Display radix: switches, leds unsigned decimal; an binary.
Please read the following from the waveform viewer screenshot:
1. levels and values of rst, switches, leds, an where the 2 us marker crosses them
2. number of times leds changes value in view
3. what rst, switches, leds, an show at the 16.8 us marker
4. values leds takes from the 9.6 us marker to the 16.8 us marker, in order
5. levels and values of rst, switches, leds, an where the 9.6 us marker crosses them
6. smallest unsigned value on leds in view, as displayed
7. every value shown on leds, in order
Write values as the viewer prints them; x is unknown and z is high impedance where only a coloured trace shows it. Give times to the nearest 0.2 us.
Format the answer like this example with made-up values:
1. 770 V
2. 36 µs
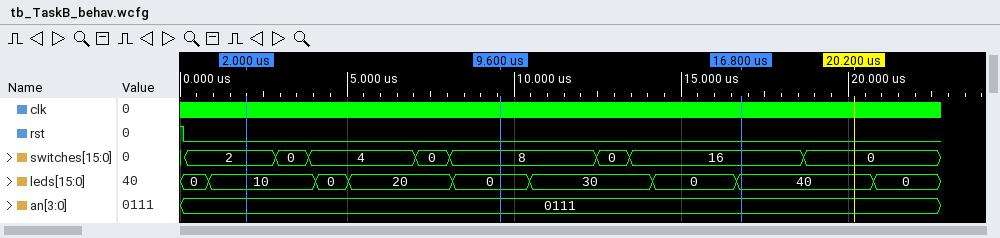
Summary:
1. rst=0, switches=2, leds=10, an=0111
2. 8
3. rst=0, switches=16, leds=40, an=0111
4. 0, 30, 0, 40
5. rst=0, switches=8, leds=0, an=0111
6. 0
7. 0, 10, 0, 20, 0, 30, 0, 40, 0
